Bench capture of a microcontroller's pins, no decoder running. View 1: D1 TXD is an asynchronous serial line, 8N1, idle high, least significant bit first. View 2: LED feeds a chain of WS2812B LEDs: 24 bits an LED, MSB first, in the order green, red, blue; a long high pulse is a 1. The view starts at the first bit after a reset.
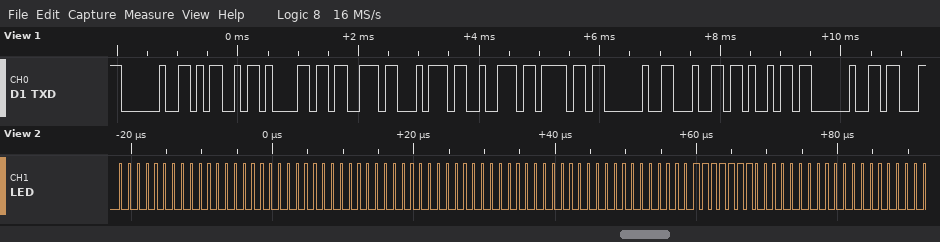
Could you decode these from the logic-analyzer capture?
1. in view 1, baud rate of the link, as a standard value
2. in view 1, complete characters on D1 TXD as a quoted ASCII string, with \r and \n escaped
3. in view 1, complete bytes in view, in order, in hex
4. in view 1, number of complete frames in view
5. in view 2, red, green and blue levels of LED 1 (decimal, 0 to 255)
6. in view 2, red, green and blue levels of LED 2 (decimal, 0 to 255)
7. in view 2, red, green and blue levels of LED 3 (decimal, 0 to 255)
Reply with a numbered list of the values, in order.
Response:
1. 9600 baud
2. " Mastro di "
3. 20 4D 61 73 74 72 6F 20 64 69 20
4. 11
5. 0, 0, 0
6. 0, 0, 0
7. 0, 0, 127
